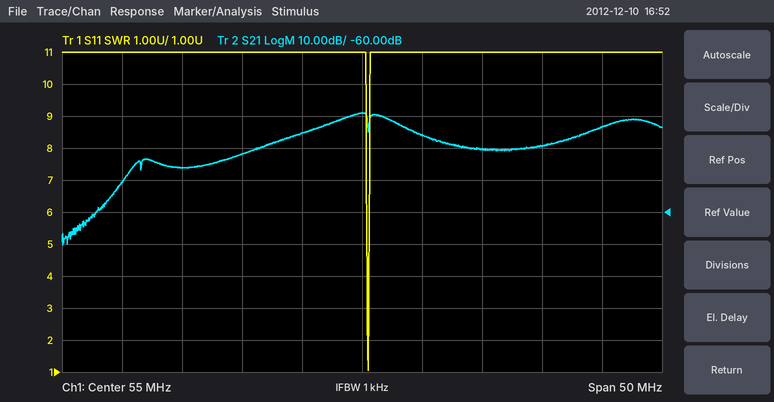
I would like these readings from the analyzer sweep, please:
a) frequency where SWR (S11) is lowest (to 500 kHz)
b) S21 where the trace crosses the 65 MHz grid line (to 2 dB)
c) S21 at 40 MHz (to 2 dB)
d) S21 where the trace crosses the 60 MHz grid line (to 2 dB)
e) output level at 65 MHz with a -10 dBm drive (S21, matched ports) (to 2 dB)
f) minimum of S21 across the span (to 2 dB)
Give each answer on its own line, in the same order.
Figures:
55.5 MHz
-40 dB
-46 dB
-36 dB
-50 dBm
-70 dB
